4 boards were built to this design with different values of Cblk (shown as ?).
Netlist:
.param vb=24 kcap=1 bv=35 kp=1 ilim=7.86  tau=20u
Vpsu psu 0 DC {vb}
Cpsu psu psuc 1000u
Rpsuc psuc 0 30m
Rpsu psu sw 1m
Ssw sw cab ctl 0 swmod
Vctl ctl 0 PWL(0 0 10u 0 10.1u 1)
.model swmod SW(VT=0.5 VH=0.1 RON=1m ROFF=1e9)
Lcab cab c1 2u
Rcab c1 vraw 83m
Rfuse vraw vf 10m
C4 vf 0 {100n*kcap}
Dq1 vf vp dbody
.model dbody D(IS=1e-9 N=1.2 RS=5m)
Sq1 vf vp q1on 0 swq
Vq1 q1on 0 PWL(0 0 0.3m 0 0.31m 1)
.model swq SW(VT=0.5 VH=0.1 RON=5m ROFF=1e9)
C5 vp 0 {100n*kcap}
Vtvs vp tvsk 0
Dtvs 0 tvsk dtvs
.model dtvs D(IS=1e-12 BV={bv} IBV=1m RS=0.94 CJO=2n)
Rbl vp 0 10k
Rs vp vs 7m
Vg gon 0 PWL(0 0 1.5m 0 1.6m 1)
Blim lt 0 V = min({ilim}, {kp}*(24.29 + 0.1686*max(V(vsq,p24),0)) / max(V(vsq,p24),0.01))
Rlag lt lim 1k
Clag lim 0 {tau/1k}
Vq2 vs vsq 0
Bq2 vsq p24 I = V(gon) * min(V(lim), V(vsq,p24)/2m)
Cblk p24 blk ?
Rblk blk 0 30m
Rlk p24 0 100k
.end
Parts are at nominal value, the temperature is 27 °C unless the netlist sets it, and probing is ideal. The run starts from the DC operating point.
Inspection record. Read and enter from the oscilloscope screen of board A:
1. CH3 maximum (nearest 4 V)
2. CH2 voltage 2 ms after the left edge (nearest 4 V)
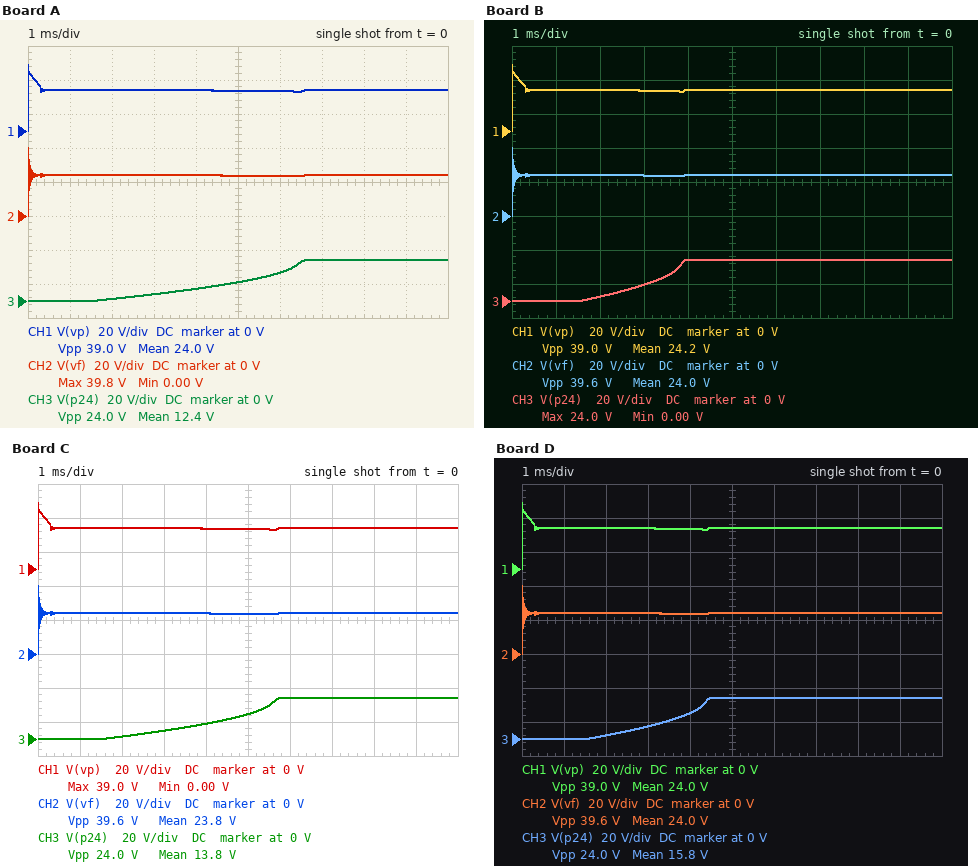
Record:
24 V
24 V
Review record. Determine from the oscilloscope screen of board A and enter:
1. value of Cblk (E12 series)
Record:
470 µF
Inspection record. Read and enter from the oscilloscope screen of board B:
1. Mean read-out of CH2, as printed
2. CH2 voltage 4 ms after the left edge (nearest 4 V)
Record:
24.0 V
24 V
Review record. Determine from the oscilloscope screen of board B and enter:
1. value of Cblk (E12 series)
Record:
220 µF
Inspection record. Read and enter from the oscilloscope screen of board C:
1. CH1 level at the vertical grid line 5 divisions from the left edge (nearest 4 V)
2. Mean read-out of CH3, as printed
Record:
24 V
13.8 V
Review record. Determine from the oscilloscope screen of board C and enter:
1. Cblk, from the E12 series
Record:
390 µF
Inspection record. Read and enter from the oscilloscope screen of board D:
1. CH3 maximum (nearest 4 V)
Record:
24 V
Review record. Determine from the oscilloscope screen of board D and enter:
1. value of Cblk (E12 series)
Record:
270 µF
